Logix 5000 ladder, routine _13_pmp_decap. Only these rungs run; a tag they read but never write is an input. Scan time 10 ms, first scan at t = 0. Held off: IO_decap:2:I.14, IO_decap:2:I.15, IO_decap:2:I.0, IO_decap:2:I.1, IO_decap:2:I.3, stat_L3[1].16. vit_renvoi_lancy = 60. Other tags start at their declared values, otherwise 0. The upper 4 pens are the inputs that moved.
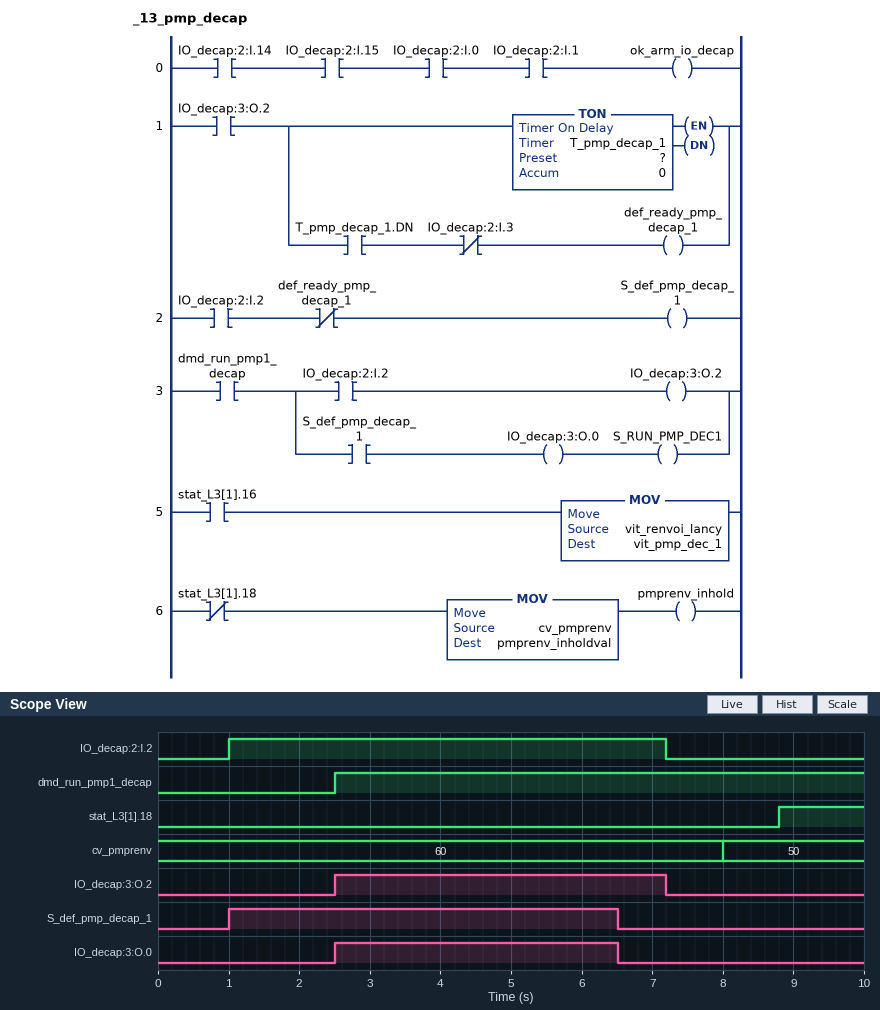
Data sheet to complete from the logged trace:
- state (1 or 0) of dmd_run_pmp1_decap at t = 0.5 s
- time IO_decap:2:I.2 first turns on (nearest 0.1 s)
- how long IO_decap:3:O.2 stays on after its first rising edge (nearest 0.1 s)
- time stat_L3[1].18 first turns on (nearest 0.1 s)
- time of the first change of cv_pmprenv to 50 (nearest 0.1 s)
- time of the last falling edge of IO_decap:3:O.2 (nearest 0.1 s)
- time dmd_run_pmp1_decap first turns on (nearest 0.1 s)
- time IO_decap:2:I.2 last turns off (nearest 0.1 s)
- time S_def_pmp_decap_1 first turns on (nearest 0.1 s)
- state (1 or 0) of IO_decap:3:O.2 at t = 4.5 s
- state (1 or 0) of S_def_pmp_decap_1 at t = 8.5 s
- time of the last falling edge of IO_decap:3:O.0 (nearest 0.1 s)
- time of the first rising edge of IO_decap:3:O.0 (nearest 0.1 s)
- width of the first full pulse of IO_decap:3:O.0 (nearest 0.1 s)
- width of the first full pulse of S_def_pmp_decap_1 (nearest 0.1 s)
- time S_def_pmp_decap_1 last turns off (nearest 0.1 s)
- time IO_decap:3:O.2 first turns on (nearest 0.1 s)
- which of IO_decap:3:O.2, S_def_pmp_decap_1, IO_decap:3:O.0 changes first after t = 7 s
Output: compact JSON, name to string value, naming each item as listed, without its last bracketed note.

{"state (1 or 0) of dmd_run_pmp1_decap at t = 0.5 s": "0", "time IO_decap:2:I.2 first turns on": "1.0 s", "how long IO_decap:3:O.2 stays on after its first rising edge": "4.7 s", "time stat_L3[1].18 first turns on": "8.8 s", "time of the first change of cv_pmprenv to 50": "8.0 s", "time of the last falling edge of IO_decap:3:O.2": "7.2 s", "time dmd_run_pmp1_decap first turns on": "2.5 s", "time IO_decap:2:I.2 last turns off": "7.2 s", "time S_def_pmp_decap_1 first turns on": "1.0 s", "state (1 or 0) of IO_decap:3:O.2 at t = 4.5 s": "1", "state (1 or 0) of S_def_pmp_decap_1 at t = 8.5 s": "0", "time of the last falling edge of IO_decap:3:O.0": "6.5 s", "time of the first rising edge of IO_decap:3:O.0": "2.5 s", "width of the first full pulse of IO_decap:3:O.0": "4.0 s", "width of the first full pulse of S_def_pmp_decap_1": "5.5 s", "time S_def_pmp_decap_1 last turns off": "6.5 s", "time IO_decap:3:O.2 first turns on": "2.5 s", "which of IO_decap:3:O.2, S_def_pmp_decap_1, IO_decap:3:O.0 changes first after t = 7 s": "IO_decap:3:O.2"}
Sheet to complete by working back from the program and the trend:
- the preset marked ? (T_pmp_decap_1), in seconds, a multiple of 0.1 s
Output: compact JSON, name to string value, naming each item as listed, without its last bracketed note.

{"the preset marked ? (T_pmp_decap_1), in seconds, a multiple of 0.1 s": "4.0 s"}
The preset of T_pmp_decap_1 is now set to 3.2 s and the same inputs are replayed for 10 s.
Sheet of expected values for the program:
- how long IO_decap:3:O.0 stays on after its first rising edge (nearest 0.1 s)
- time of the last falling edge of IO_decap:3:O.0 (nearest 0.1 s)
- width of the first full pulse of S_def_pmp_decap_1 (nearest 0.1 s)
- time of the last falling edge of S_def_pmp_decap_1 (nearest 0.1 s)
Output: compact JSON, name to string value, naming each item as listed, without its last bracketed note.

{"how long IO_decap:3:O.0 stays on after its first rising edge": "3.2 s", "time of the last falling edge of IO_decap:3:O.0": "5.7 s", "width of the first full pulse of S_def_pmp_decap_1": "4.7 s", "time of the last falling edge of S_def_pmp_decap_1": "5.7 s"}
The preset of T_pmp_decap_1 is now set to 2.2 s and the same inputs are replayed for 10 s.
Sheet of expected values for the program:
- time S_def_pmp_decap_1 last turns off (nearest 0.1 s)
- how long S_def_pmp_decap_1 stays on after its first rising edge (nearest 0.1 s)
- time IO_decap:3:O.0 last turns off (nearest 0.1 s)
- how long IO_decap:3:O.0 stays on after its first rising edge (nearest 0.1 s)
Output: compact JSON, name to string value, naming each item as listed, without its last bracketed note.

{"time S_def_pmp_decap_1 last turns off": "4.7 s", "how long S_def_pmp_decap_1 stays on after its first rising edge": "3.7 s", "time IO_decap:3:O.0 last turns off": "4.7 s", "how long IO_decap:3:O.0 stays on after its first rising edge": "2.2 s"}
